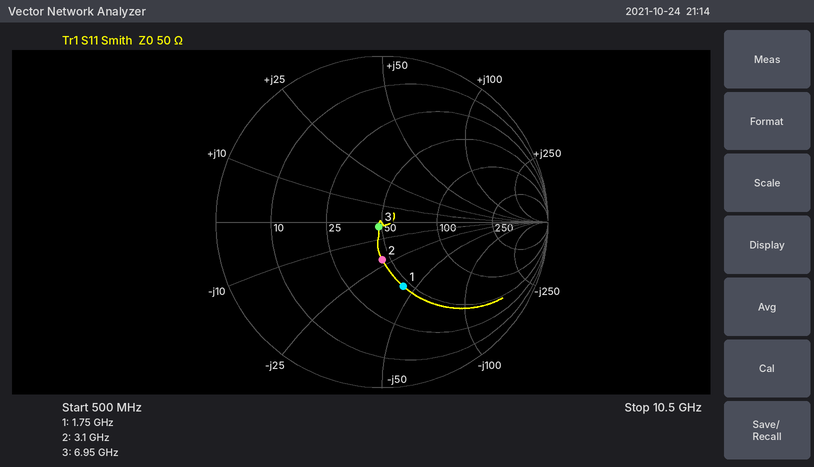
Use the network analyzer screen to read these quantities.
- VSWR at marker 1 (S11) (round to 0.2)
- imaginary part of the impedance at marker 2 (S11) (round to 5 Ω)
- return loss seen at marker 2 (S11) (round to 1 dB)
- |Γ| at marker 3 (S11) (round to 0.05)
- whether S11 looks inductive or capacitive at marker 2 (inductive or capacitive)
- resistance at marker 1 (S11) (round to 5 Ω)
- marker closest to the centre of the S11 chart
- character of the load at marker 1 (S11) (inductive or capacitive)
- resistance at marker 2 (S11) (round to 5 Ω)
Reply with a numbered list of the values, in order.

1. 2.4
2. -20 Ω
3. 13 dB
4. 0.05
5. capacitive
6. 45 Ω
7. marker 3
8. capacitive
9. 45 Ω
